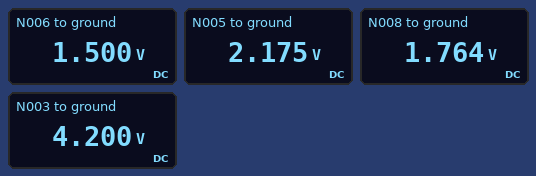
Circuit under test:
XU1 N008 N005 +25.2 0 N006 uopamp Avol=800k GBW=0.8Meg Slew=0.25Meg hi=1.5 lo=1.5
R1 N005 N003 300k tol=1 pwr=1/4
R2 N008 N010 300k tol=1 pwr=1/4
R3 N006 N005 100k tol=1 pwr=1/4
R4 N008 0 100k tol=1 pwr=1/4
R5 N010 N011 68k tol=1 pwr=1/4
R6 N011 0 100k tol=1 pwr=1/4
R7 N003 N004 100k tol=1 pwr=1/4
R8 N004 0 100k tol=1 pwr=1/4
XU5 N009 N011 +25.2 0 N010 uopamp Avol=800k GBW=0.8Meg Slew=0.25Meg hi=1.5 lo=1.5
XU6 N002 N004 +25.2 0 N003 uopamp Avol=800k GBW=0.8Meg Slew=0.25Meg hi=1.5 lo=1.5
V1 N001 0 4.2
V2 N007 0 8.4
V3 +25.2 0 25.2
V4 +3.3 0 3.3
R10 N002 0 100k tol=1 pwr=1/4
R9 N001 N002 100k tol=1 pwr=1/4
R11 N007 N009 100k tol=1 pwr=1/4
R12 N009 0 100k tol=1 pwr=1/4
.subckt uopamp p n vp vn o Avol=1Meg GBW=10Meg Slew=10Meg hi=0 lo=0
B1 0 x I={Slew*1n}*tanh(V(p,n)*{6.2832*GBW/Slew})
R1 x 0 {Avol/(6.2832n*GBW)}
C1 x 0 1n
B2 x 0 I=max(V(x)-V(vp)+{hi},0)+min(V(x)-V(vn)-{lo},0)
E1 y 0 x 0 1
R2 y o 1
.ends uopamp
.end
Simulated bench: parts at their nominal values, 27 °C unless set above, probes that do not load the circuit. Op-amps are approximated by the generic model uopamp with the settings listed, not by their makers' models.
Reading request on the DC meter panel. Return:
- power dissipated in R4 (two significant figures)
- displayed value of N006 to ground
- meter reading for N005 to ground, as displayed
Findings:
31 µW
1.500 V
2.175 V
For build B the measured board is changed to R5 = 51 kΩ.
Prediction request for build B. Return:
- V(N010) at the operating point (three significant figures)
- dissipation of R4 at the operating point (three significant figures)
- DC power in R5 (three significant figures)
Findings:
6.34 V
25.1 µW
90.0 µW
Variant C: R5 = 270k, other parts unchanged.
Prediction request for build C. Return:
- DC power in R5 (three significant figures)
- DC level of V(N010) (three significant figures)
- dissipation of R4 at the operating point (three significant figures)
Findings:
476 µW
15.5 V
151 µW
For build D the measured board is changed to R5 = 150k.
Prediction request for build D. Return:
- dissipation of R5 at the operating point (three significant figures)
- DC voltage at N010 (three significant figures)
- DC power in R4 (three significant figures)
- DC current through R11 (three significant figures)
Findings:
265 µW
10.5 V
68.9 µW
42.0 µA
